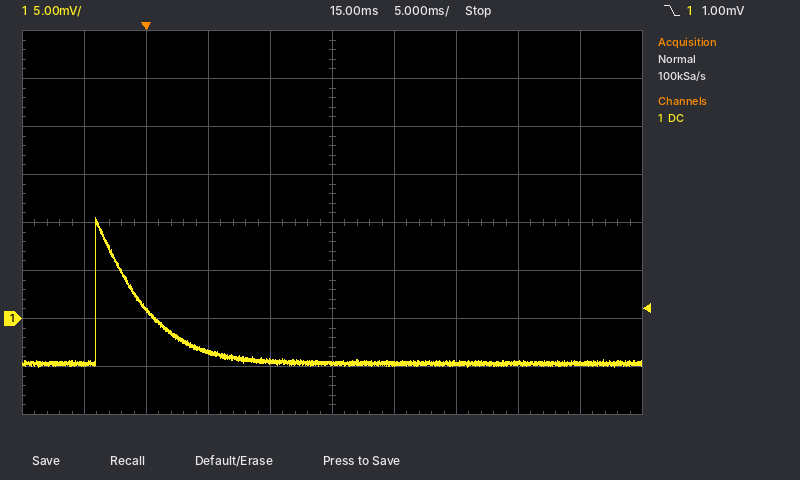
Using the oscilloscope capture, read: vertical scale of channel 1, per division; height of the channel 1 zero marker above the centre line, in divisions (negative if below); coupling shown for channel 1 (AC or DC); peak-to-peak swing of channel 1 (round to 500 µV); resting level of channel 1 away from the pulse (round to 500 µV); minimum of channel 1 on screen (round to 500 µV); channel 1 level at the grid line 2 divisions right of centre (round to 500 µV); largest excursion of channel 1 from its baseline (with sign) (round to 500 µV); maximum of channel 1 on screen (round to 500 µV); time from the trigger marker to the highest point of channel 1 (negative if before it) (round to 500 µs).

5 mV
-2.0 div
DC
15.5 mV
-4.5 mV
-5.0 mV
-4.5 mV
+15.0 mV
10.5 mV
-4.0 ms
